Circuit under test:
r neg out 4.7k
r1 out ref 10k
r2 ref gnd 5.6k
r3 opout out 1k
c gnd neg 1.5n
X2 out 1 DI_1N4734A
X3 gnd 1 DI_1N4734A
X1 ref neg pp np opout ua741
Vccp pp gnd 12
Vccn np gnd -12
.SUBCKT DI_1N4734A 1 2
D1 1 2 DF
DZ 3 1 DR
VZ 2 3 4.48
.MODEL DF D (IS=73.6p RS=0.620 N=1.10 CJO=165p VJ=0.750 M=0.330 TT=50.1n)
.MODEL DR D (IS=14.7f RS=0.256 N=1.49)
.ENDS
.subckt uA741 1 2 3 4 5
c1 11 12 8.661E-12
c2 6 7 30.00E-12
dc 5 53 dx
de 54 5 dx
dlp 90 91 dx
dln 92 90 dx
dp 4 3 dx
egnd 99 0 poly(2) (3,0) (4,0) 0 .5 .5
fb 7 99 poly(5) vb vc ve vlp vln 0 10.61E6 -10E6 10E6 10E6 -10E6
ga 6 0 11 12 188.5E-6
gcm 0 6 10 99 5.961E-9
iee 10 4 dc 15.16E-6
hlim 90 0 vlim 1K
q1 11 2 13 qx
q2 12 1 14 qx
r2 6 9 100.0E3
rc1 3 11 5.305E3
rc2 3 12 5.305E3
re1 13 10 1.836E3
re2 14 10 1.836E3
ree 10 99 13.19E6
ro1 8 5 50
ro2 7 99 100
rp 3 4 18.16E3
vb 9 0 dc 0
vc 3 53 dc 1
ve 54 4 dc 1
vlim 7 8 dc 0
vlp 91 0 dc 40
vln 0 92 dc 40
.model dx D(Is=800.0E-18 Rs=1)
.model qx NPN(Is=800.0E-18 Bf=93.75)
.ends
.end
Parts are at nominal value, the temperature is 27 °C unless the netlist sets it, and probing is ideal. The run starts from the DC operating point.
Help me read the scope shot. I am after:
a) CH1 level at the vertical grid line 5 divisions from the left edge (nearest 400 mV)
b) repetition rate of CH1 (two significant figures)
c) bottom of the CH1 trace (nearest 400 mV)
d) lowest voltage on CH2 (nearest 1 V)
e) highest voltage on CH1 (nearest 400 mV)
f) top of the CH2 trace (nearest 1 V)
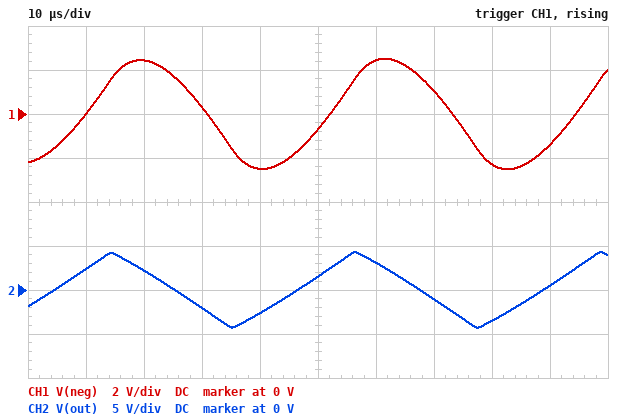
-800 mV
24 kHz
-2.4 V
-4 V
2.4 V
4 V
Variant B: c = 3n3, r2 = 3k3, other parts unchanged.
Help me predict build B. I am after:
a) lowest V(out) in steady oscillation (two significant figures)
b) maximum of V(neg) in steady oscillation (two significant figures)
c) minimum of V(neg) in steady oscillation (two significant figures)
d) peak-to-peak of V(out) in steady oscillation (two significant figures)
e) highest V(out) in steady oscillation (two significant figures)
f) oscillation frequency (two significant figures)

-5.9 V
3.0 V
-3.0 V
12 V
5.9 V
15 kHz
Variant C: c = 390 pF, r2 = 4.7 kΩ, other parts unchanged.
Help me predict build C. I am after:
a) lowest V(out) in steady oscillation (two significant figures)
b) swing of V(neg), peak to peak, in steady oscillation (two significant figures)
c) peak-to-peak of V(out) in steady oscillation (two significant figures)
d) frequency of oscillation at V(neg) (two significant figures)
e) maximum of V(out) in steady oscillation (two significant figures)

-990 mV
1.2 V
2.0 V
96 kHz
990 mV
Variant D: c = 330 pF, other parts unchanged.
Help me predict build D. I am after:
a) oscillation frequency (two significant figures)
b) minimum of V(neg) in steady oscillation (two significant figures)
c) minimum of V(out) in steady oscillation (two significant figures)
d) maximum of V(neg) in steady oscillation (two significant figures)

100 kHz
-580 mV
-920 mV
580 mV
